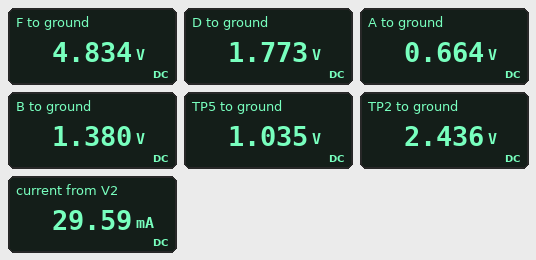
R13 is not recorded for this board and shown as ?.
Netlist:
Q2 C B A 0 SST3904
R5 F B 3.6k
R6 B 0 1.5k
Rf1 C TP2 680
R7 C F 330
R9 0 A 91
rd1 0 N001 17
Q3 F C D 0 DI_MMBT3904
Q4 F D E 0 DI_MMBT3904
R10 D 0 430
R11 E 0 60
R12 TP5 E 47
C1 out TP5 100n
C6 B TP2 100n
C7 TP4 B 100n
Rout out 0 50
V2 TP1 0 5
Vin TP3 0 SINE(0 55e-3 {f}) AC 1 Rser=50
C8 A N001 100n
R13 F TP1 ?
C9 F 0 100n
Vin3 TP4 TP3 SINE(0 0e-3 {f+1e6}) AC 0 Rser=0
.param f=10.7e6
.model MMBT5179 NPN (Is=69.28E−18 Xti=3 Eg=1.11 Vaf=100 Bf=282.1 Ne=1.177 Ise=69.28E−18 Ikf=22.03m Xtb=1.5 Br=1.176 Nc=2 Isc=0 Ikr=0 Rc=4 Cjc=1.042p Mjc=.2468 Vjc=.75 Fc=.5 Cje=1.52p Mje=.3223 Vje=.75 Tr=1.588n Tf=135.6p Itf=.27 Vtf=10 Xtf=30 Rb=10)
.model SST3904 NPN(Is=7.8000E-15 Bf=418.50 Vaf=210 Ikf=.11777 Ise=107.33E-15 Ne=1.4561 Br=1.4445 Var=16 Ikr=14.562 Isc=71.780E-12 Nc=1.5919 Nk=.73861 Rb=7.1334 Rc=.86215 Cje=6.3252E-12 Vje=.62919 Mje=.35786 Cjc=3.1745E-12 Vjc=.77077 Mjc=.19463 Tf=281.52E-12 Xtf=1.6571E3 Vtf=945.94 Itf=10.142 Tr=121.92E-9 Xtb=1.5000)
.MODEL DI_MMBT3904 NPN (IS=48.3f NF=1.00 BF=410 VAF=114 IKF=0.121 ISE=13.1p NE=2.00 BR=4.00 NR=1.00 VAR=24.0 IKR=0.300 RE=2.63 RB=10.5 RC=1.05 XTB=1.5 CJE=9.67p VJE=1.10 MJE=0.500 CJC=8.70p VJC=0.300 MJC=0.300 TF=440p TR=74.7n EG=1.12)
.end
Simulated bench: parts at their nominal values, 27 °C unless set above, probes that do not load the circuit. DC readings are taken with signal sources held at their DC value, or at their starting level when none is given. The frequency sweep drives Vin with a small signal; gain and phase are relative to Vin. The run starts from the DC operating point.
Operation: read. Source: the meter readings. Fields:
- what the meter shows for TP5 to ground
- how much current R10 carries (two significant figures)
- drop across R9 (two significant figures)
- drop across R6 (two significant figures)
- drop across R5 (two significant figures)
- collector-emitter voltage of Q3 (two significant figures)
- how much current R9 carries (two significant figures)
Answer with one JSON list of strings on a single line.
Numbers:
["1.035 V", "4.1 mA", "660 mV", "1.4 V", "3.5 V", "3.1 V", "7.3 mA"]
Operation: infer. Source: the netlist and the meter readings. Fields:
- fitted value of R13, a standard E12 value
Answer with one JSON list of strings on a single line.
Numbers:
["5.6 Ω"]
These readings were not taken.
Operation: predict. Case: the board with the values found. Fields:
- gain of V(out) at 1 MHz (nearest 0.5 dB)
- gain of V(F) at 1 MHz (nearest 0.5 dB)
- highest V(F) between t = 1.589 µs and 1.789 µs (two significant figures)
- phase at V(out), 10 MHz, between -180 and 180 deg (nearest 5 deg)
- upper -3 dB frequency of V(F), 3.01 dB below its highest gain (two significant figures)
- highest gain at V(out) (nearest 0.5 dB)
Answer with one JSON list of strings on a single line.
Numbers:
["8.5 dB", "-14.0 dB", "4.8 V", "170 deg", "400 kHz", "8.5 dB"]
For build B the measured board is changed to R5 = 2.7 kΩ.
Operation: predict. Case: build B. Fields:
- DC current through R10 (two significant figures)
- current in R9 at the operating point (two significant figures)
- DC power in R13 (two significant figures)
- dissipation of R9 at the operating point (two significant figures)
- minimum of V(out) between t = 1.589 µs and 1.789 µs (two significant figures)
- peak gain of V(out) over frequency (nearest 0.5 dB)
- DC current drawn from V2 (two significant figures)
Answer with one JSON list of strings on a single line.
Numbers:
["1.8 mA", "11 mA", "1.4 mW", "10 mW", "-45 mV", "6.5 dB", "16 mA"]
